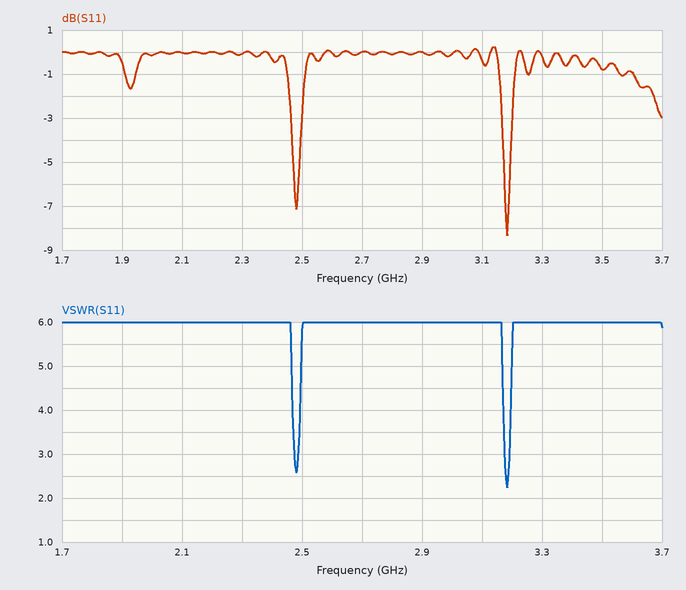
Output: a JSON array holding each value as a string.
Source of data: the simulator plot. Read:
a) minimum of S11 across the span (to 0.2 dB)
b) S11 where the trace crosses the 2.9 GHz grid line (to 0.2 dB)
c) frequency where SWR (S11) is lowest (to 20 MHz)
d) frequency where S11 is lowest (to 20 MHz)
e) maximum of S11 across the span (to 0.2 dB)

["-8.4 dB", "0.0 dB", "3.18 GHz", "3.18 GHz", "0.2 dB"]
